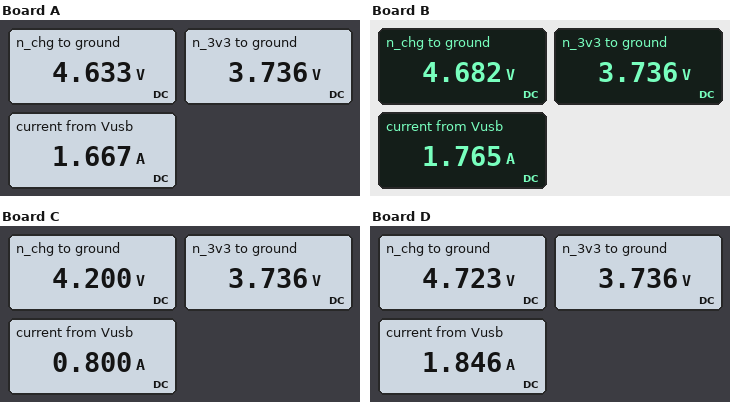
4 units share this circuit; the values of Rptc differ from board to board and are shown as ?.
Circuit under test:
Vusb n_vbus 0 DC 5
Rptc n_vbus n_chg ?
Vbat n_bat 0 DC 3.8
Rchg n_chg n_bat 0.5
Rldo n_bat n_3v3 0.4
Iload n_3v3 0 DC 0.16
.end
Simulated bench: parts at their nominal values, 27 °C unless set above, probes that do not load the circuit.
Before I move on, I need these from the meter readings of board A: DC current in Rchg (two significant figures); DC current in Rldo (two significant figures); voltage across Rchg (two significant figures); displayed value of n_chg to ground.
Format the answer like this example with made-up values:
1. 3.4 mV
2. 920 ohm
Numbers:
1. 1.7 A
2. 160 mA
3. 830 mV
4. 4.633 V
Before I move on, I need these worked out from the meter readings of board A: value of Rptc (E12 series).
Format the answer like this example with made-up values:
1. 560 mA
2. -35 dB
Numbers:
1. 0.22 Ω
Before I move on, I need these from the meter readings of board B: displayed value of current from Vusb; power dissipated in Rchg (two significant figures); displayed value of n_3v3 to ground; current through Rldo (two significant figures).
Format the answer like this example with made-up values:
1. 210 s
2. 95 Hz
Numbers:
1. 1.765 A
2. 1.6 W
3. 3.736 V
4. 160 mA
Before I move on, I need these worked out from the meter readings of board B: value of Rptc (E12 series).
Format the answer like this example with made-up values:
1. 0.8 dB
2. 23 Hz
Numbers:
1. 0.18 Ω
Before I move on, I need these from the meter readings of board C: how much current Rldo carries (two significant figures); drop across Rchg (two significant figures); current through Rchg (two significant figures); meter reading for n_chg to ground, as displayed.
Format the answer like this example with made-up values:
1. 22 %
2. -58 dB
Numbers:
1. 160 mA
2. 400 mV
3. 800 mA
4. 4.200 V
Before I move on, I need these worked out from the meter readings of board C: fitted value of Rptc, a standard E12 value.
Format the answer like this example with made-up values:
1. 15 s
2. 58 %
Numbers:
1. 1 Ω
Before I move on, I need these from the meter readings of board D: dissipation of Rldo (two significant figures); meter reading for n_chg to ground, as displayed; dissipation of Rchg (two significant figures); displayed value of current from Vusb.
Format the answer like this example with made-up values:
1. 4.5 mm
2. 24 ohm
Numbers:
1. 10 mW
2. 4.723 V
3. 1.7 W
4. 1.846 A
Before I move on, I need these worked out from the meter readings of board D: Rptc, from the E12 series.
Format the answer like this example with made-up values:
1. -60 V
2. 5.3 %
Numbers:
1. 0.15 Ω
